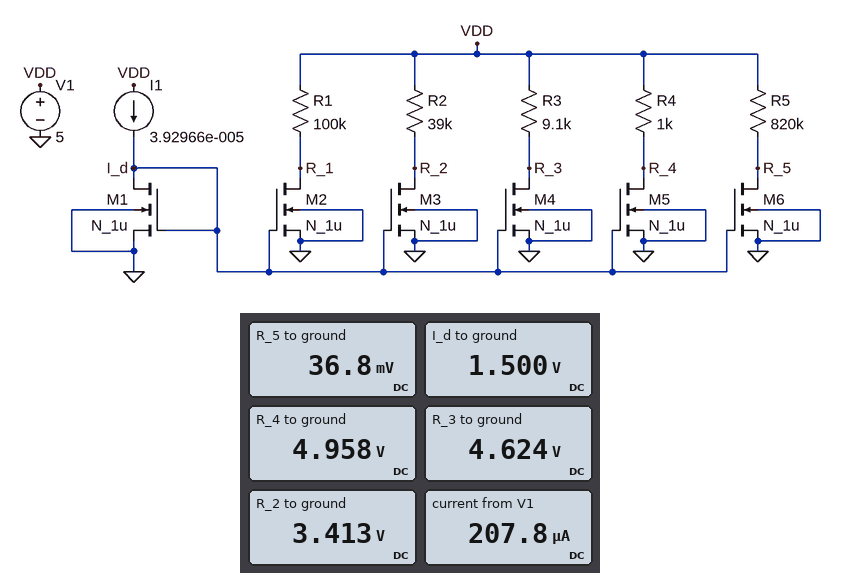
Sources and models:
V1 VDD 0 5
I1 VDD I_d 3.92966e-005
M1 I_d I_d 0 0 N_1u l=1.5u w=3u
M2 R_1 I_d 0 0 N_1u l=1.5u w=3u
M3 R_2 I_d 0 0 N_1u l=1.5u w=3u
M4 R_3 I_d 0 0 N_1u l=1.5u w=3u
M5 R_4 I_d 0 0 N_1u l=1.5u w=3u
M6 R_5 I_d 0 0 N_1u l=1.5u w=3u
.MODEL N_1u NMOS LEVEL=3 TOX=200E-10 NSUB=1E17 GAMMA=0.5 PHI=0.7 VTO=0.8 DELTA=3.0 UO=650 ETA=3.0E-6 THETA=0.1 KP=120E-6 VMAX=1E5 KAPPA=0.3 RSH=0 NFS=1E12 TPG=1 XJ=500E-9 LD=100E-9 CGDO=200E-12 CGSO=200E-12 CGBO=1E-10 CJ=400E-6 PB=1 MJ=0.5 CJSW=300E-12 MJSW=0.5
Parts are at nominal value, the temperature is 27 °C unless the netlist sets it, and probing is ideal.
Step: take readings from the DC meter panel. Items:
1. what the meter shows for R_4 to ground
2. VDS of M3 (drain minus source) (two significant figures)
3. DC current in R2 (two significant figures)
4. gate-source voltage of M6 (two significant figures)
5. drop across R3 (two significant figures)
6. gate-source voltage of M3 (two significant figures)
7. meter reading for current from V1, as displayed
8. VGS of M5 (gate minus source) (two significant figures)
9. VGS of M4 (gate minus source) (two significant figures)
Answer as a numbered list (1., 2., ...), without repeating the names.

1. 4.958 V
2. 3.4 V
3. 41 µA
4. 1.5 V
5. 380 mV
6. 1.5 V
7. 207.8 µA
8. 1.5 V
9. 1.5 V
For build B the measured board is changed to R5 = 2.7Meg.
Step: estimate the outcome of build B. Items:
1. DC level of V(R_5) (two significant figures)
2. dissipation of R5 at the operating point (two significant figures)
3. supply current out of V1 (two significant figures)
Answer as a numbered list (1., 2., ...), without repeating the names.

1. 11 mV
2. 9.2 µW
3. 200 µA
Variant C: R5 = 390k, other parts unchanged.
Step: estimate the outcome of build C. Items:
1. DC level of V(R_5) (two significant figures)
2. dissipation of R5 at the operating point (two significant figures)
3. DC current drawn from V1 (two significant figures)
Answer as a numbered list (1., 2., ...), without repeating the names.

1. 82 mV
2. 62 µW
3. 210 µA
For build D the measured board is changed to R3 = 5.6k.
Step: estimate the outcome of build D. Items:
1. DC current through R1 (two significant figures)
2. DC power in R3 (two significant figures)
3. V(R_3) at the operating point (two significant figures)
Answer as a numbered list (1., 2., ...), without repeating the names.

1. 39 µA
2. 9.6 µW
3. 4.8 V
